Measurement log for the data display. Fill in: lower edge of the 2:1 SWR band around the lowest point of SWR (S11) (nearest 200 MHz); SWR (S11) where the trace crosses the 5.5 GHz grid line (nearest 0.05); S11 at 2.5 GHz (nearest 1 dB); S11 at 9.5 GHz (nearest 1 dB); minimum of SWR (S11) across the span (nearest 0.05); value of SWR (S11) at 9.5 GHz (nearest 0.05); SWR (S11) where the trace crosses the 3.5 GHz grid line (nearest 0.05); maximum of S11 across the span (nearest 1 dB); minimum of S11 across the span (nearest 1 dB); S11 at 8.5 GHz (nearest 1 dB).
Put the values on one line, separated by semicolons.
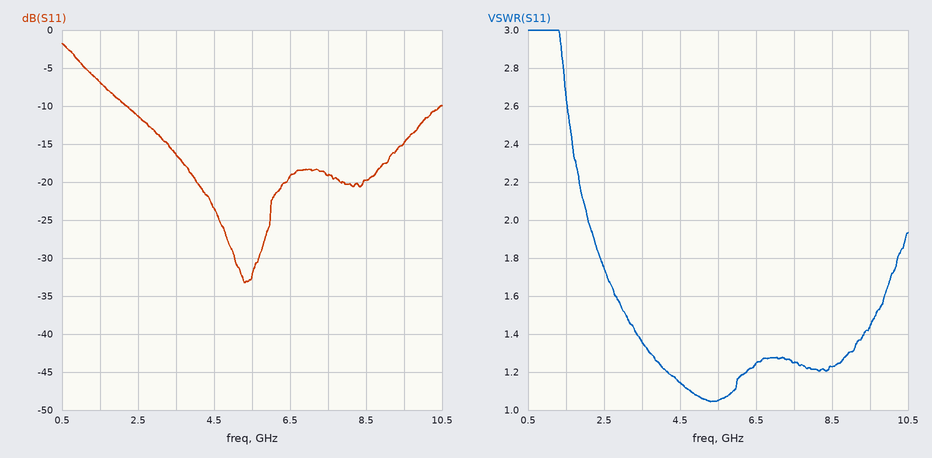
2.0 GHz; 1.05; -11 dB; -15 dB; 1.05; 1.45; 1.35; -2 dB; -33 dB; -20 dB
